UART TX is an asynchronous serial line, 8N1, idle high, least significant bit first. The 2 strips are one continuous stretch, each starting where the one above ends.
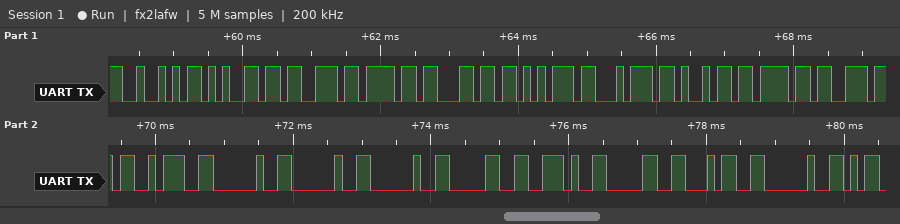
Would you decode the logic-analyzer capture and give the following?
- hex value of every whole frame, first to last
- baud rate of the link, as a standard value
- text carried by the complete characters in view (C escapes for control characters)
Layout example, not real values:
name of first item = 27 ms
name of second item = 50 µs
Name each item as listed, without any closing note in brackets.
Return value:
hex value of every whole frame, first to last = 0x52 0x65 0x73 0x6F 0x6C 0x75 0x74 0x69 0x6F 0x6E 0x3A 0x20 0x20 0x20 0x30 0x2E 0x30 0x34 0x20
baud rate of the link, as a standard value = 9600 baud
text carried by the complete characters in view = "Resolution:   0.04 "
